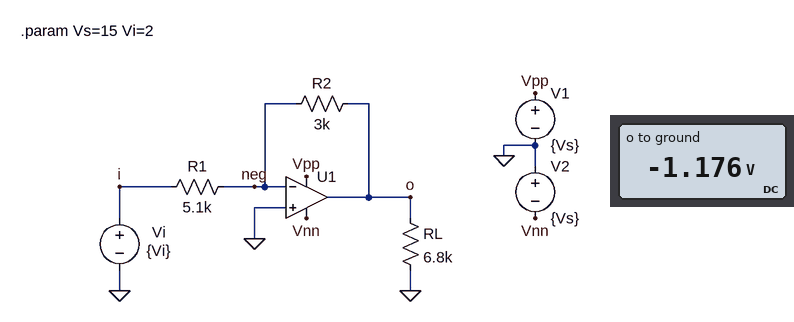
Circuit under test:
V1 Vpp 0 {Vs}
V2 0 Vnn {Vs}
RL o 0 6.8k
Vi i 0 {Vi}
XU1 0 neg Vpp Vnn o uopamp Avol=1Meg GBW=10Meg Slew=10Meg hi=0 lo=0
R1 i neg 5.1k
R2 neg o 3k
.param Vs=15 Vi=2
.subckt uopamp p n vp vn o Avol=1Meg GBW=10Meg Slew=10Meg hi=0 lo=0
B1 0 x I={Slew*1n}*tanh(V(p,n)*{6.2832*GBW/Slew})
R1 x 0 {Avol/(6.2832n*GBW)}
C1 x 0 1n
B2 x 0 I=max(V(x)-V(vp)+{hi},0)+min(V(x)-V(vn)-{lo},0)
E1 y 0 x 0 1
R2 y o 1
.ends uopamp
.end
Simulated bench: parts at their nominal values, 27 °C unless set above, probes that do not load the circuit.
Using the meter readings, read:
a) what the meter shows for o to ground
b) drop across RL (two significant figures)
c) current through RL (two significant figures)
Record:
-1.176 V
1.2 V
170 µA
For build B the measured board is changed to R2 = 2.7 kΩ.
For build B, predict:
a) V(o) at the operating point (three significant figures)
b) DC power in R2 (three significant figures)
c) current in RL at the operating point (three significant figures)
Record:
-1.06 V
415 µW
156 µA
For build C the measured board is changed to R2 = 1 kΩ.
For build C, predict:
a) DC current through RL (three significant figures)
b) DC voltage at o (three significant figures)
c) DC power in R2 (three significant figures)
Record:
57.7 µA
-392 mV
154 µW
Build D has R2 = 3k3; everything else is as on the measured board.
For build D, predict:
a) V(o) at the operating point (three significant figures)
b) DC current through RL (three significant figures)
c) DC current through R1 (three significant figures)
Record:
-1.29 V
190 µA
392 µA
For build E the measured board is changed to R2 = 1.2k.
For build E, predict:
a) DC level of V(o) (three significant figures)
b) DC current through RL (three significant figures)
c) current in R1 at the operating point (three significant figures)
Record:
-471 mV
69.2 µA
392 µA
